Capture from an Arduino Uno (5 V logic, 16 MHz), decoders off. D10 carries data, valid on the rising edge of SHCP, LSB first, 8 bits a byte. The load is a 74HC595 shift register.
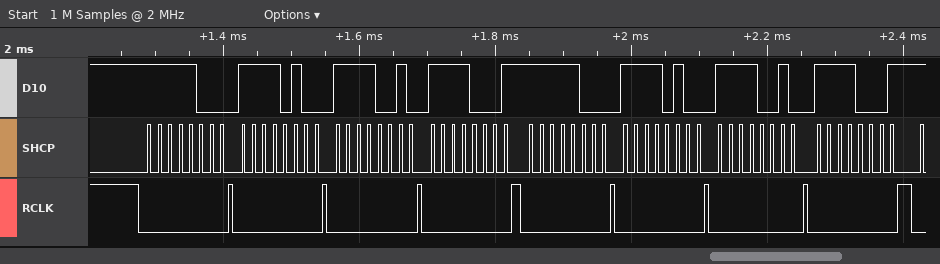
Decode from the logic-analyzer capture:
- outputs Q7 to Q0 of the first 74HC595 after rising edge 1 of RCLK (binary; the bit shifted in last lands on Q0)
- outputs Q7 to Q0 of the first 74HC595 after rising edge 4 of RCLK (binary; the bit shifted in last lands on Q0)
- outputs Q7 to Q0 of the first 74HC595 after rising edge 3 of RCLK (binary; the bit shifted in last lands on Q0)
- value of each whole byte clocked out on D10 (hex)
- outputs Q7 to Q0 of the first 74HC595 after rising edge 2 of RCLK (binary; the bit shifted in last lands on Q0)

11111000
11110001
11110010
0x1F 0x2F 0x4F 0x8F 0x1F 0x2F 0x4F 0x8F
11110100
